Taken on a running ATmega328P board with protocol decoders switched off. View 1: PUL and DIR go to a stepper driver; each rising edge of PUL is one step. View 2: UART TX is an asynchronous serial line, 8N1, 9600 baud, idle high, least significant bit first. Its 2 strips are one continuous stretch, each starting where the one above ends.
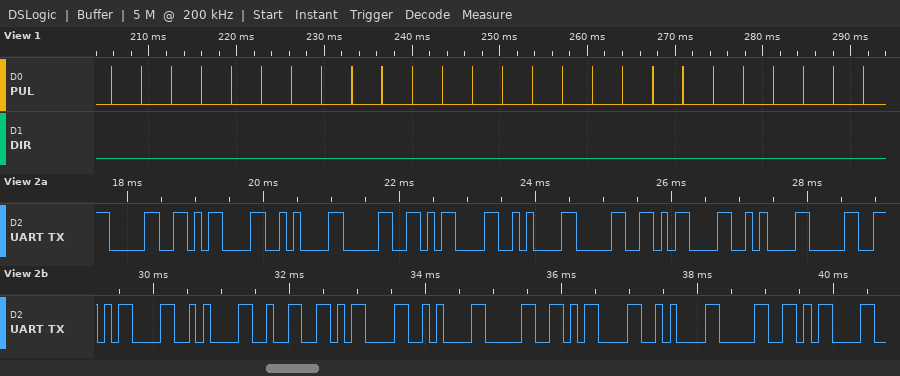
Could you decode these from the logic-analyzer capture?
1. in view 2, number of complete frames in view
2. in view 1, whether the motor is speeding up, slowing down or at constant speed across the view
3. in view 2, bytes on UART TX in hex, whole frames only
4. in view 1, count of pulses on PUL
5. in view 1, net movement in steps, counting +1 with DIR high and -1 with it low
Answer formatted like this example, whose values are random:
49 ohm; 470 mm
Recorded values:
20; constant speed; 30 0D 0A 30 0D 0A 30 0D 0A 30 0D 0A 32 0D 0A 30 0D 0A 30 0D; 26; -26
